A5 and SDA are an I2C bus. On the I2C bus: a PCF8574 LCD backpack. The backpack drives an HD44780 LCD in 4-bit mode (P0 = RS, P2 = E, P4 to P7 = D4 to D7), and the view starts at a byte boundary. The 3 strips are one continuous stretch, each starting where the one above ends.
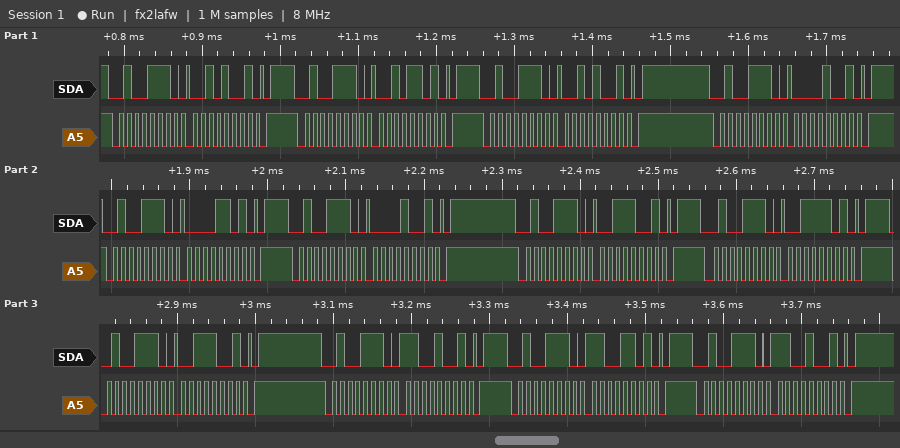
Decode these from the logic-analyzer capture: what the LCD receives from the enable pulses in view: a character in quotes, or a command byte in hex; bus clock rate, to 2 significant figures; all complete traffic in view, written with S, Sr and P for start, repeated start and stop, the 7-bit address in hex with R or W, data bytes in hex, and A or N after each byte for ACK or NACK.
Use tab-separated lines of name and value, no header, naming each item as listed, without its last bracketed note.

what the LCD receives from the enable pulses in view: a character in quotes, or a command byte in hex	' ' '<'
bus clock rate, to 2 significant figures	100 kHz
all complete traffic in view, written with S, Sr and P for start, repeated start and stop, the 7-bit address in hex with R or W, data bytes in hex, and A or N after each byte for ACK or NACK	S 27W A 29 A P S 27W A 2D A P S 27W A 29 A P S 27W A 09 A P S 27W A 0D A P S 27W A 09 A P S 27W A 39 A P S 27W A 3D A P S 27W A 39 A P S 27W A C9 A P S 27W A CD A P S 27W A C9 A P
